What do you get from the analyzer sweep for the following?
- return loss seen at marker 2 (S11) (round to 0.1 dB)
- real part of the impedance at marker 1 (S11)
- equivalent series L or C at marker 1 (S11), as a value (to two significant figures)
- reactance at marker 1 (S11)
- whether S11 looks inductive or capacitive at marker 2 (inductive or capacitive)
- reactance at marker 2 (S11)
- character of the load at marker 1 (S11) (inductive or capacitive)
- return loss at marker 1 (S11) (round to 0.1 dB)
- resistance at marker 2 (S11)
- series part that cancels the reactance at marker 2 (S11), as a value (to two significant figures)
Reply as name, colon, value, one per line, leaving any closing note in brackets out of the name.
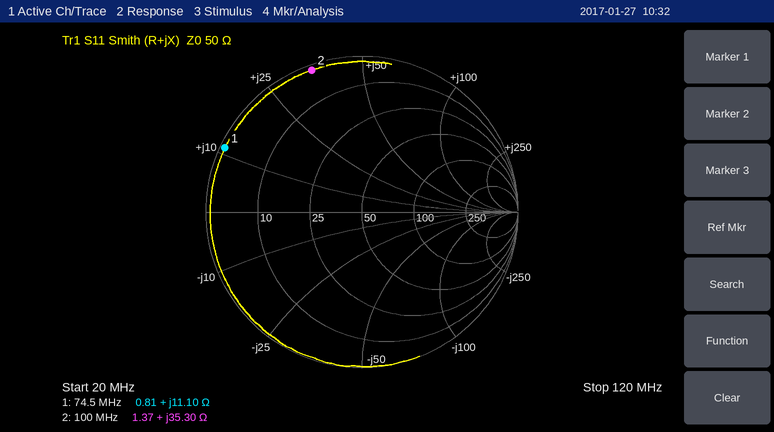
return loss seen at marker 2 (S11): 0.3 dB
real part of the impedance at marker 1: 0.81 Ω
equivalent series L or C at marker 1 (S11), as a value: 24 nH
reactance at marker 1: +11.10 Ω
whether S11 looks inductive or capacitive at marker 2: inductive
reactance at marker 2: +35.30 Ω
character of the load at marker 1 (S11): inductive
return loss at marker 1 (S11): 0.3 dB
resistance at marker 2: 1.37 Ω
series part that cancels the reactance at marker 2 (S11), as a value: 45 pF
